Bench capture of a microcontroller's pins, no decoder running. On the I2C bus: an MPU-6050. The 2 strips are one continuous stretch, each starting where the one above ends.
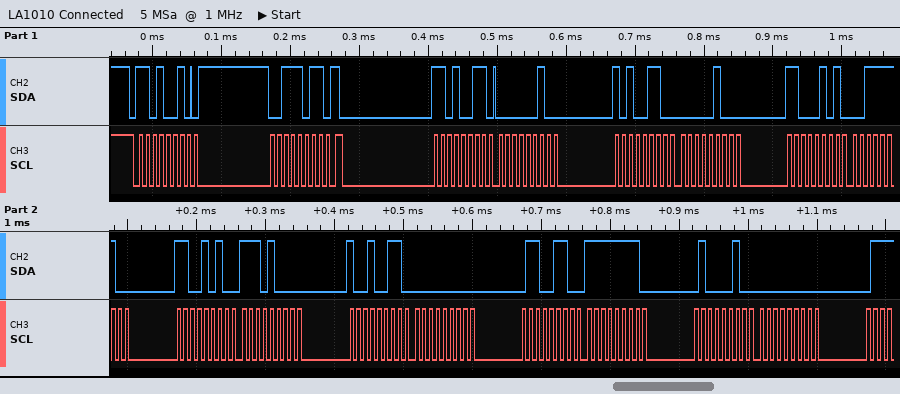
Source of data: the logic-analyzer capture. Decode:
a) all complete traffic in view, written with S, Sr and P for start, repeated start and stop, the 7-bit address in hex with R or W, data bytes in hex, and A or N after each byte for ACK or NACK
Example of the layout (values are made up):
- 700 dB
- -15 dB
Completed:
- S 69W A 3B A Sr 69R A 02 A A6 A 04 A C5 A 3E A CA A E8 A 93 A 00 A 66 A FF A 42 A 00 A
